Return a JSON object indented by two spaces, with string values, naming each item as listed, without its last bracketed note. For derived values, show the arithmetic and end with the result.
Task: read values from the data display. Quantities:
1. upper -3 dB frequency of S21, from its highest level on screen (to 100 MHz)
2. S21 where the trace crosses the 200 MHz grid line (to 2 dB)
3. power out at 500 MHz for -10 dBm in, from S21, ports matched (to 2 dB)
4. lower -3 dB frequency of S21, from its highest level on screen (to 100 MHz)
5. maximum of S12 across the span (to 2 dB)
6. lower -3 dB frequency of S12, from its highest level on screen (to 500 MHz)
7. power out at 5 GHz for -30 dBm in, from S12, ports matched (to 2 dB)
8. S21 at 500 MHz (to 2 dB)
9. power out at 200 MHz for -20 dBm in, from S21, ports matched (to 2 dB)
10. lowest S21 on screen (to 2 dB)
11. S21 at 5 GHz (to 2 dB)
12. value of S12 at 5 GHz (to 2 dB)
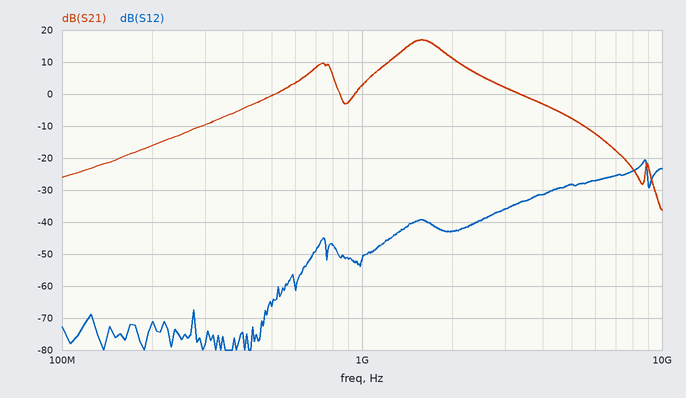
{
  "upper -3 dB frequency of S21, from its highest level on screen": "1.8 GHz",
  "S21 where the trace crosses the 200 MHz grid line": "-16 dB",
  "power out at 500 MHz for -10 dBm in, from S21, ports matched": "-10 dBm + (0 dB) = -10 dBm",
  "lower -3 dB frequency of S21, from its highest level on screen": "1.4 GHz",
  "maximum of S12 across the span": "-20 dB",
  "lower -3 dB frequency of S12, from its highest level on screen": "8.0 GHz",
  "power out at 5 GHz for -30 dBm in, from S12, ports matched": "-30 dBm + (-28 dB) = -58 dBm",
  "S21 at 500 MHz": "0 dB",
  "power out at 200 MHz for -20 dBm in, from S21, ports matched": "-20 dBm + (-16 dB) = -36 dBm",
  "lowest S21 on screen": "-36 dB",
  "S21 at 5 GHz": "-8 dB",
  "value of S12 at 5 GHz": "-28 dB"
}
